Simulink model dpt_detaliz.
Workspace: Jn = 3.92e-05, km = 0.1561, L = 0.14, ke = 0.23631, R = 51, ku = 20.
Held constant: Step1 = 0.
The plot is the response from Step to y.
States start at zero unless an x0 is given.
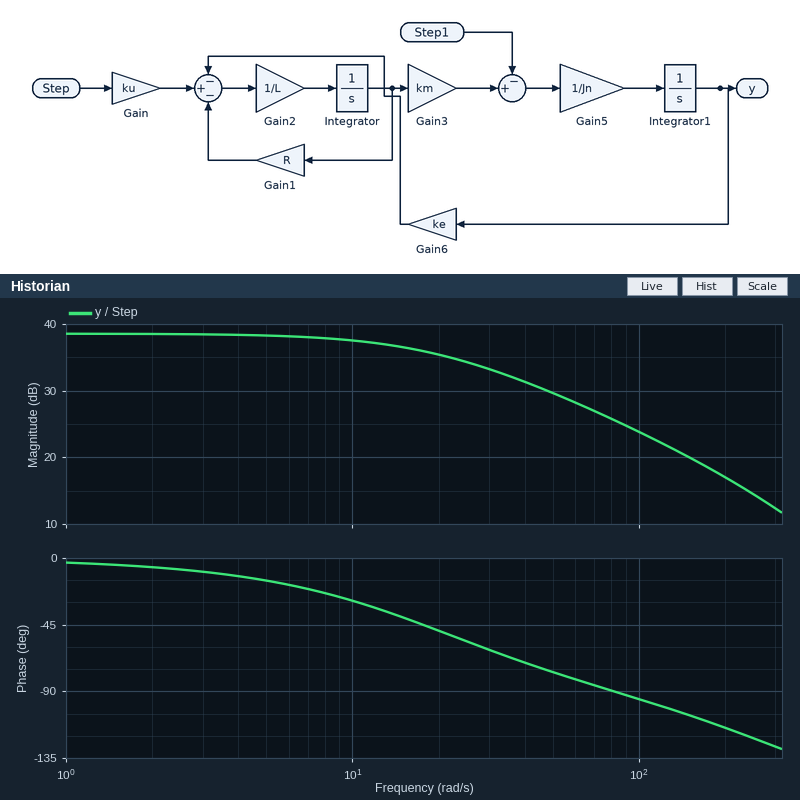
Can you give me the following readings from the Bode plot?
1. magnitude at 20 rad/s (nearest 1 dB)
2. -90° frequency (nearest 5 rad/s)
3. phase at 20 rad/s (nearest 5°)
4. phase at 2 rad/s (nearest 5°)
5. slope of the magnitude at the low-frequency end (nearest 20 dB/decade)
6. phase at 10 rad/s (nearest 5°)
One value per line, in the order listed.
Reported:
35 dB
80 rad/s
-50°
-5°
0 dB/decade
-30°
